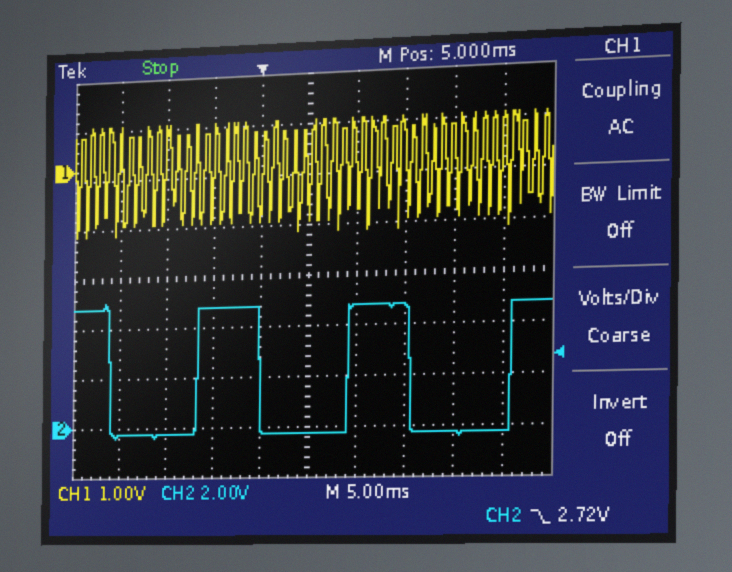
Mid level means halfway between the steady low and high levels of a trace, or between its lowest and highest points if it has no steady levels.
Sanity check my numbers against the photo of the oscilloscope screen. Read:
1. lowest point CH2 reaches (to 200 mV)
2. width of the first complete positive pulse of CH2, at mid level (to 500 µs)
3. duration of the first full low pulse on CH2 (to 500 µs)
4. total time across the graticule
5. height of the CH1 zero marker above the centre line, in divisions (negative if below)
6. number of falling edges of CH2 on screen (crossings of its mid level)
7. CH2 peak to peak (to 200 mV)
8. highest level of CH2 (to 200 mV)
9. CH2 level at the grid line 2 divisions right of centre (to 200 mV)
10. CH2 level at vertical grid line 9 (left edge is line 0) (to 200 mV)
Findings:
-400 mV
6.5 ms
9.5 ms
50 ms
+2.2 div
3
5.4 V
5.0 V
4.8 V
-200 mV
